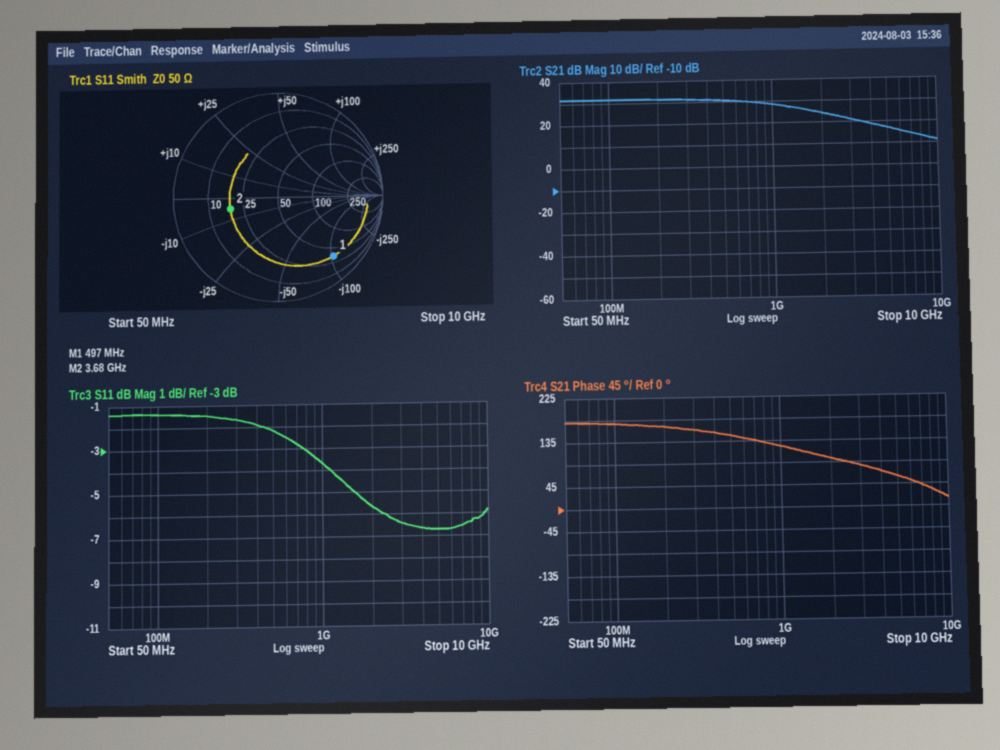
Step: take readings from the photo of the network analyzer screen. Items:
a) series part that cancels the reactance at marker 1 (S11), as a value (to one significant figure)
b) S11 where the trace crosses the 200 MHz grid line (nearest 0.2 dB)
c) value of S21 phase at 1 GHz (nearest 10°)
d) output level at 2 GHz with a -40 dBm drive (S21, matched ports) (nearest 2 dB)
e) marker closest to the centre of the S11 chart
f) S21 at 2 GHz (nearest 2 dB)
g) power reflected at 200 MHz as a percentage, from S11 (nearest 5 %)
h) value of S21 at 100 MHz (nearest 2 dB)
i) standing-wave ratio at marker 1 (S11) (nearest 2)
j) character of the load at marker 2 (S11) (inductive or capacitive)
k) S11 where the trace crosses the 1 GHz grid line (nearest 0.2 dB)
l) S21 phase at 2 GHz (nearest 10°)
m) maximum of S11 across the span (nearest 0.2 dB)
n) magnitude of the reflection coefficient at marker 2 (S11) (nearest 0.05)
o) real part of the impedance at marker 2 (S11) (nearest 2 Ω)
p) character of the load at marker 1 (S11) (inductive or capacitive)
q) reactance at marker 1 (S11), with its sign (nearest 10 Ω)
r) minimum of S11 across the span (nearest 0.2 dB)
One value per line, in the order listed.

30 nH
-1.4 dB
120°
-16 dBm
marker 2
24 dB
70 %
32 dB
8
capacitive
-3.6 dB
100°
-1.4 dB
0.45
18 Ω
capacitive
-100 Ω
-6.8 dB
